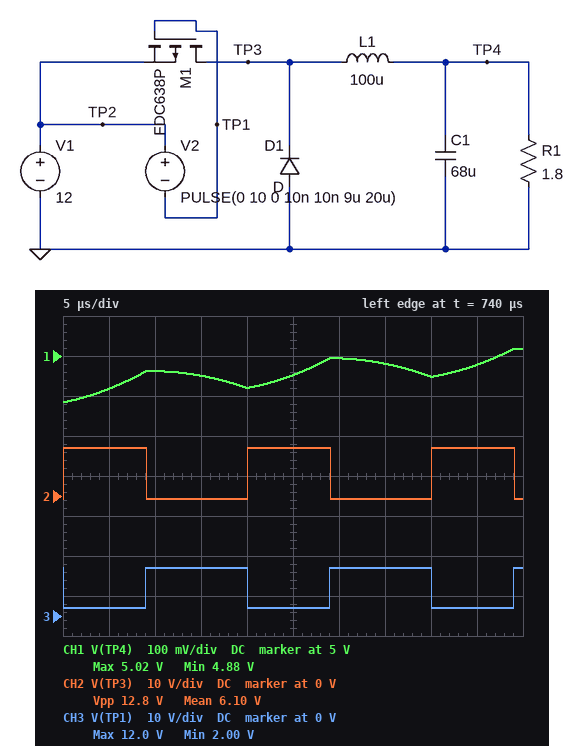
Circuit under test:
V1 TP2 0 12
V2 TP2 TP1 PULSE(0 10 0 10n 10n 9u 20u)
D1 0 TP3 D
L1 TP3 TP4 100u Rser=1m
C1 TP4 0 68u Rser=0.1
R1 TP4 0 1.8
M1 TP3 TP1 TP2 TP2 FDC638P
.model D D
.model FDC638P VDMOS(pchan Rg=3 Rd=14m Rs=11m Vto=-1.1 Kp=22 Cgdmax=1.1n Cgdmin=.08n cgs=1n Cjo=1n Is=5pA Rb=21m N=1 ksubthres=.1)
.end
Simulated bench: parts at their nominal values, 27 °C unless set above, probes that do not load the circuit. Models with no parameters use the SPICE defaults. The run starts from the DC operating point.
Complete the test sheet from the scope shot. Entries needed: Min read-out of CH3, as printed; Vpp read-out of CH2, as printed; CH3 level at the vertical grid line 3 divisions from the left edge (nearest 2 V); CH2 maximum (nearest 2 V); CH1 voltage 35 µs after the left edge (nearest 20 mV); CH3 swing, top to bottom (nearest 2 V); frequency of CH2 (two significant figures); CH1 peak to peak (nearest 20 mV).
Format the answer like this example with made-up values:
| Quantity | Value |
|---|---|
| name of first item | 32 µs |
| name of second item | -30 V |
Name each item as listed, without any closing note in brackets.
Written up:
| Quantity | Value |
|---|---|
| Min read-out of CH3, as printed | 2.00 V |
| Vpp read-out of CH2, as printed | 12.8 V |
| CH3 level at the vertical grid line 3 divisions from the left edge | 12 V |
| CH2 maximum | 12 V |
| CH1 voltage 35 µs after the left edge | 4.98 V |
| CH3 swing, top to bottom | 10 V |
| frequency of CH2 | 50 kHz |
| CH1 peak to peak | 140 mV |
